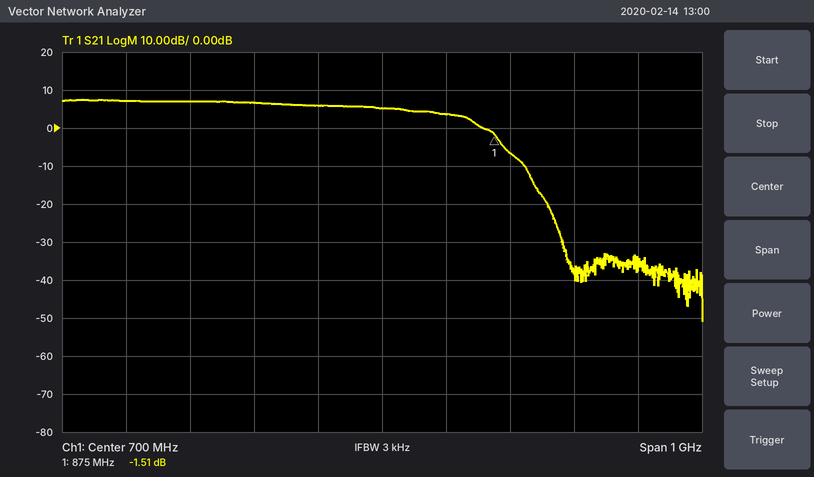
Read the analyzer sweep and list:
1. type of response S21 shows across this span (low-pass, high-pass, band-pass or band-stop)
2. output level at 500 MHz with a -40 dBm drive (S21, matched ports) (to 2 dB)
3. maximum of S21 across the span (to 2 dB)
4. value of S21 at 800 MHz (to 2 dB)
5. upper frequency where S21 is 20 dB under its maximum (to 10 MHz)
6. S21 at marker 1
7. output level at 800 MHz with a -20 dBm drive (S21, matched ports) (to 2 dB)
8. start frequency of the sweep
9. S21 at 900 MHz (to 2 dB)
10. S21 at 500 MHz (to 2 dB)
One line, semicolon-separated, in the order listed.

low-pass; -34 dBm; 8 dB; 4 dB; 930 MHz; -1.51 dB; -16 dBm; 200 MHz; -6 dB; 6 dB
